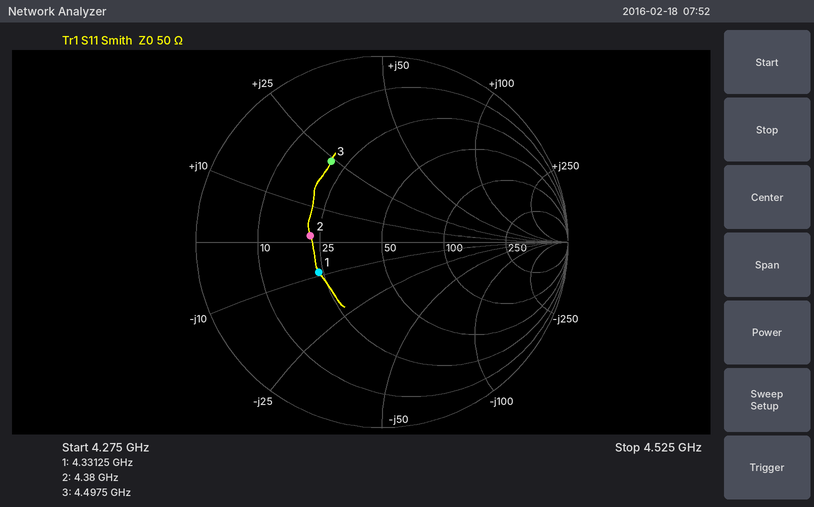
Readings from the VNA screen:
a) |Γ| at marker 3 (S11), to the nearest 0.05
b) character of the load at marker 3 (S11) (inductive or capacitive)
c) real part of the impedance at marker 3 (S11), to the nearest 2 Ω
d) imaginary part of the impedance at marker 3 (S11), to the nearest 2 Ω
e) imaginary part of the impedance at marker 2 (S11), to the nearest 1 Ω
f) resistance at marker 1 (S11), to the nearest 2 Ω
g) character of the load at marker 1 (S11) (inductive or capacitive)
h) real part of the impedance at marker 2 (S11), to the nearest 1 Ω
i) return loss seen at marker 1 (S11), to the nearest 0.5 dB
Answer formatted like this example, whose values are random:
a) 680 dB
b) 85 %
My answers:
a) 0.50
b) inductive
c) 20 Ω
d) +24 Ω
e) +2 Ω
f) 24 Ω
g) capacitive
h) 22 Ω
i) 8.5 dB
